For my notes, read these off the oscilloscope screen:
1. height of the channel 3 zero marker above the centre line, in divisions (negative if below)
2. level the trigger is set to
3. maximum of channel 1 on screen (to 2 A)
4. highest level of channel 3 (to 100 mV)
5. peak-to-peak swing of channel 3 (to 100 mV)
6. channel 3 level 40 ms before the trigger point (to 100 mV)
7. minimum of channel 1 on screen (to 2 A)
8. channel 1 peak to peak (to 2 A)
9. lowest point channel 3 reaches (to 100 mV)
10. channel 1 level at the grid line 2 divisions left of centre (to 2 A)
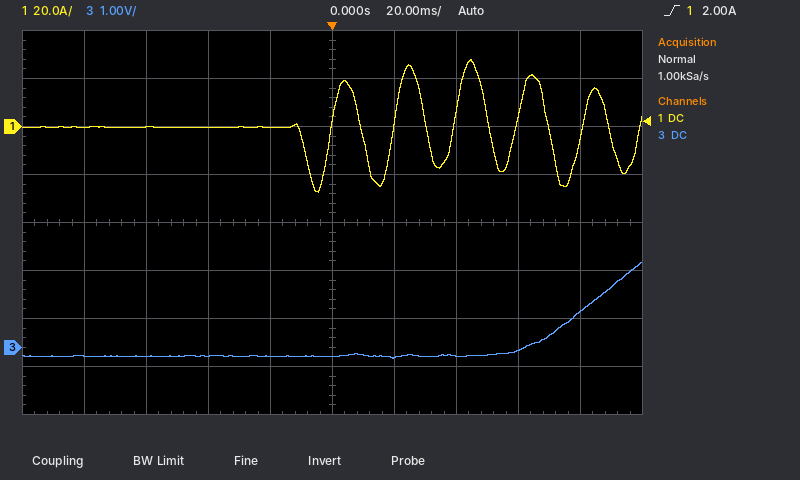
-2.6 div
2.00 A
28 A
1.8 V
2.0 V
-200 mV
-28 A
56 A
-200 mV
0 A
